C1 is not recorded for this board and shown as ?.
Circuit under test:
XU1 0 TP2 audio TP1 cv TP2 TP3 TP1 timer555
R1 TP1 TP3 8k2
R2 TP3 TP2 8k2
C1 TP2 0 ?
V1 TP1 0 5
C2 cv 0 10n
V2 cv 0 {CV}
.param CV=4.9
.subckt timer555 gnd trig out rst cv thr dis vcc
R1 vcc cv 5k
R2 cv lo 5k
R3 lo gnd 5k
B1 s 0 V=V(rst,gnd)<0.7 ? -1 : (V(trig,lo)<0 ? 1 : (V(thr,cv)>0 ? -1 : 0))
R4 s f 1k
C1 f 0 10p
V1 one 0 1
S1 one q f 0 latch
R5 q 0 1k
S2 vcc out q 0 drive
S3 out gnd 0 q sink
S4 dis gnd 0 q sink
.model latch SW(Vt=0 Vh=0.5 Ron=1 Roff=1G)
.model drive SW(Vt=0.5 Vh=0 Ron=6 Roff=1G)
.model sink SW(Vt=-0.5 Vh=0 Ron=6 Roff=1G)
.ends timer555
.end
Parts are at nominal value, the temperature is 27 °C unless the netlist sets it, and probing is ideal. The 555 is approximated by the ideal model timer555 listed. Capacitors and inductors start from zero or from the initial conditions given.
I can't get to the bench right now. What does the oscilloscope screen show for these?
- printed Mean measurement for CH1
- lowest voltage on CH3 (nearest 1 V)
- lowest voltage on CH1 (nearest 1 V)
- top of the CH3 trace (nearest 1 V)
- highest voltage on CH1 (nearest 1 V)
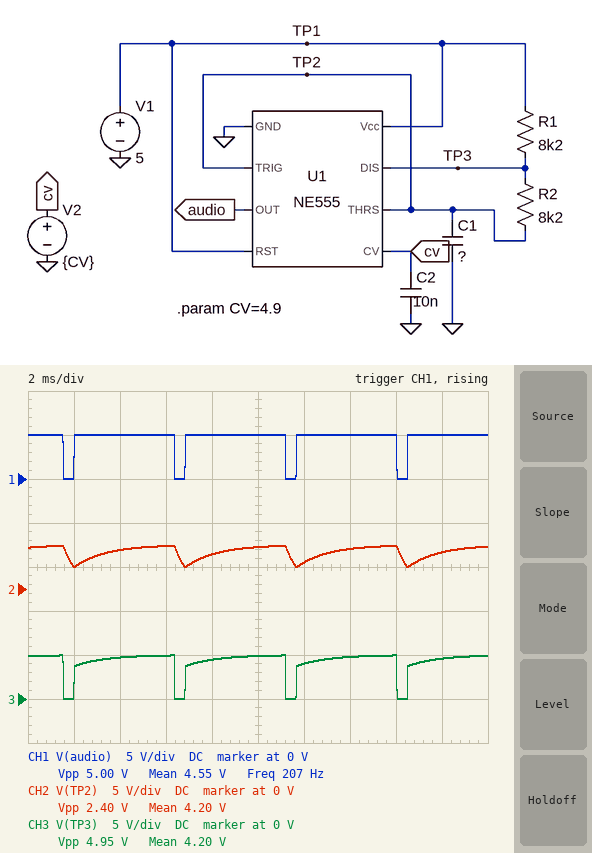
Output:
4.55 V
0 V
0 V
5 V
5 V
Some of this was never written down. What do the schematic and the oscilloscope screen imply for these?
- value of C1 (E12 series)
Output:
82 nF
